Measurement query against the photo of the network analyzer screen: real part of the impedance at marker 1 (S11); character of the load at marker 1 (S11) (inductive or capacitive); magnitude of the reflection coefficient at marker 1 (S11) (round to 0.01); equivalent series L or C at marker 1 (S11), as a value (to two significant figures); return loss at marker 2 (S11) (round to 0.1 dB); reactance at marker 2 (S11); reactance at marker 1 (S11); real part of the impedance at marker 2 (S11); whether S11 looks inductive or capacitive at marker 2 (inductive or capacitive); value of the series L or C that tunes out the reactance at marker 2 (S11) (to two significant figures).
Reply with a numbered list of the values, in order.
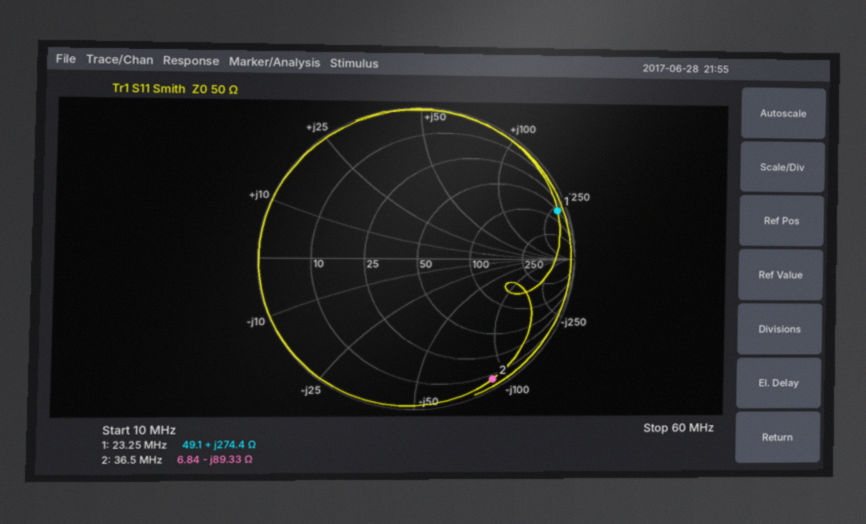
1. 49.1 Ω
2. inductive
3. 0.94
4. 1.9 µH
5. 0.6 dB
6. -89.33 Ω
7. +274.4 Ω
8. 6.84 Ω
9. capacitive
10. 390 nH
